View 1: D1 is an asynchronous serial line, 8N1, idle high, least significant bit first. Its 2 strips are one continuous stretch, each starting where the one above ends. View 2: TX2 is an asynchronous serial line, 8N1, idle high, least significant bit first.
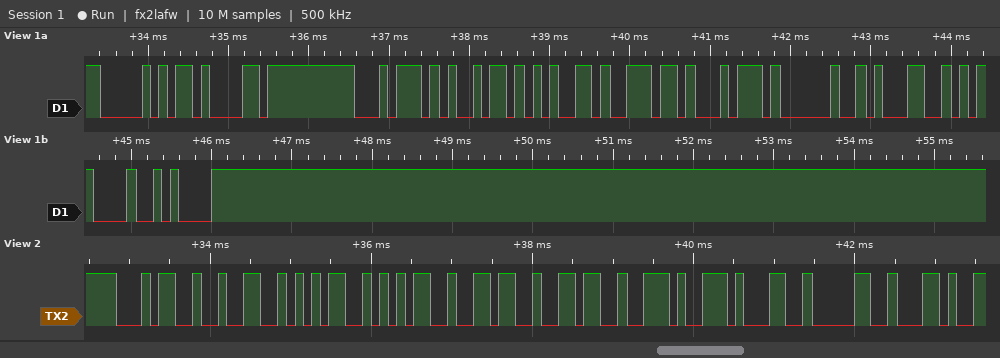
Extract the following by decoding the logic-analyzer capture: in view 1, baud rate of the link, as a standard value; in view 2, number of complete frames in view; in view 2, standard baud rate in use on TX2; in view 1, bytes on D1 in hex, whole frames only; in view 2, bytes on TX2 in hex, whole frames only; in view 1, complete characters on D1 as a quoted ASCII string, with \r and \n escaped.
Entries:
9600 baud
10
9600 baud
50 61 74 69 65 6E 74 20 31 0D 0A
34 32 35 35 36 36 2E 31 30 2C
"Patient 1\r\n"
